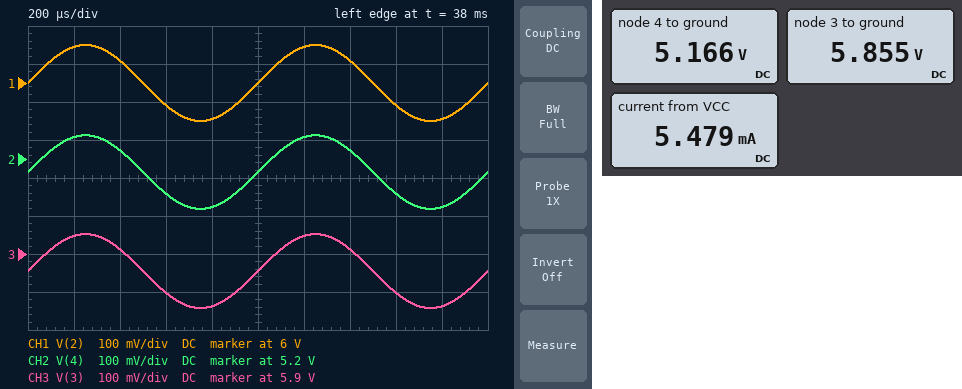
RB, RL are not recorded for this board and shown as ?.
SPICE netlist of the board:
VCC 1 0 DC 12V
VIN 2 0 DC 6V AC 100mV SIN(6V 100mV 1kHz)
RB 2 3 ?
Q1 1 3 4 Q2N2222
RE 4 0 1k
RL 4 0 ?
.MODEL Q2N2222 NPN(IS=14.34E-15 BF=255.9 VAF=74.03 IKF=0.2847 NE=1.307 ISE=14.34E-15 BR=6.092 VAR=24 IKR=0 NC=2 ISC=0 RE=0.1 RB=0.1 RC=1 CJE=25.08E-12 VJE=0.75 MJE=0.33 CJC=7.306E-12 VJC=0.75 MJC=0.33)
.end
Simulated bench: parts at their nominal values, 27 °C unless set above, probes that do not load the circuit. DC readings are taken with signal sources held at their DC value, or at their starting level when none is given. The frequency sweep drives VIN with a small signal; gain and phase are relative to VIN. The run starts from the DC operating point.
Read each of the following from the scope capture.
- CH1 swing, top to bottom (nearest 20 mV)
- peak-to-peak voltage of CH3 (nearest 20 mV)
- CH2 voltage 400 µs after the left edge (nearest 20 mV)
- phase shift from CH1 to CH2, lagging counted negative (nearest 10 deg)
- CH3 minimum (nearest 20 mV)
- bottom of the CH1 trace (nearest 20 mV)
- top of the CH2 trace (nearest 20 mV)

200 mV
200 mV
5.22 V
0 deg
5.76 V
5.90 V
5.26 V
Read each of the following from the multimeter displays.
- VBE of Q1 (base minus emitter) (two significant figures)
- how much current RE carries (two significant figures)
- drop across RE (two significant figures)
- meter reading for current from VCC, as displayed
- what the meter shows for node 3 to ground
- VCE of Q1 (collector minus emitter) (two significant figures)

690 mV
5.2 mA
5.2 V
5.479 mA
5.855 V
6.8 V
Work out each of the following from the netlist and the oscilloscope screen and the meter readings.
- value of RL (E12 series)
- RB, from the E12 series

15 kΩ
4.7 kΩ
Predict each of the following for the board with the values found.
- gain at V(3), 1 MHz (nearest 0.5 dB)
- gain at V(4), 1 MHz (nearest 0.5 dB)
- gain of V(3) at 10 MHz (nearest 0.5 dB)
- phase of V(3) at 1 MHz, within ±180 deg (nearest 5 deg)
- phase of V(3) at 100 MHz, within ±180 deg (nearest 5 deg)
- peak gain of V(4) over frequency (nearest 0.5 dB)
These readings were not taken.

-0.5 dB
-0.5 dB
-3.5 dB
-5 deg
-85 deg
-0.5 dB
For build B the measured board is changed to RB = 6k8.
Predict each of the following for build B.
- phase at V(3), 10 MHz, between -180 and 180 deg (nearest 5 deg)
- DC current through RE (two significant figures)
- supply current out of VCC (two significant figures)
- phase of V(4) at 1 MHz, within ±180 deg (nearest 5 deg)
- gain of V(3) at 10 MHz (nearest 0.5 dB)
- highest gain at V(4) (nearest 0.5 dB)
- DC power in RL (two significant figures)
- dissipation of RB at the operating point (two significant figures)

-55 deg
5.1 mA
5.4 mA
-10 deg
-5.5 dB
-0.5 dB
1.7 mW
6.3 µW
